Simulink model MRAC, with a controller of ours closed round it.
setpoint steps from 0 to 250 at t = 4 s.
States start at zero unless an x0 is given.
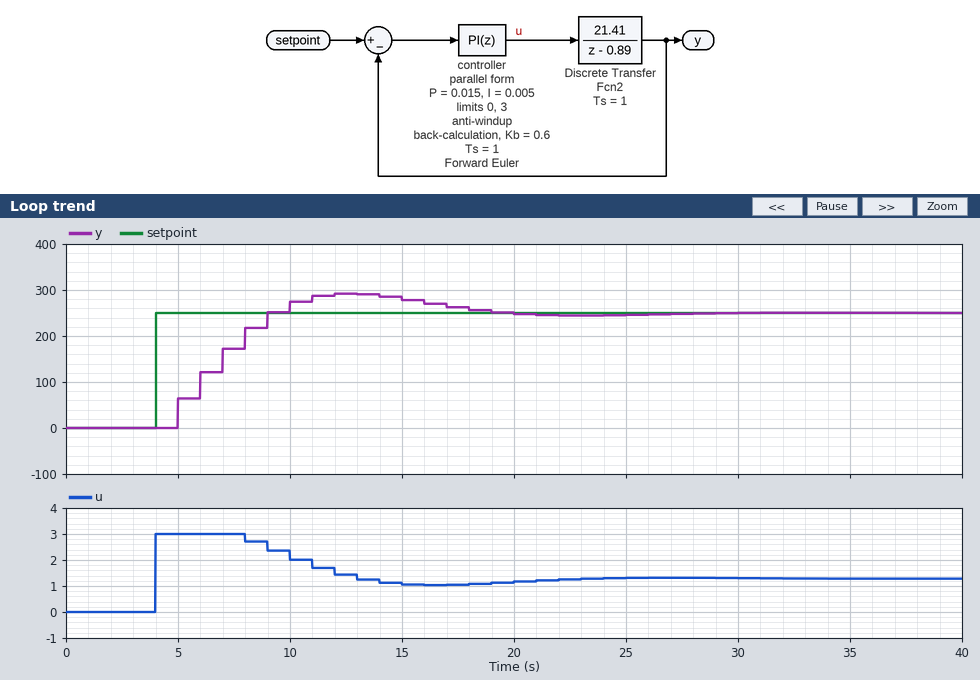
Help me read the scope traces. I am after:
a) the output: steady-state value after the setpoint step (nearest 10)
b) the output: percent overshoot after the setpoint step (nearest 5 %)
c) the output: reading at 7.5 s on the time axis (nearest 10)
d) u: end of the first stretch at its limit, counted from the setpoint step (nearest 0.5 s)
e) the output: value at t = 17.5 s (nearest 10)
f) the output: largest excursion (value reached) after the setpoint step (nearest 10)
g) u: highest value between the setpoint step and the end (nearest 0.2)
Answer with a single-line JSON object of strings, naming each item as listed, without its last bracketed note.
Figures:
{"the output: steady-state value after the setpoint step": "250", "the output: percent overshoot after the setpoint step": "15 %", "the output: reading at 7.5 s on the time axis": "170", "u: end of the first stretch at its limit, counted from the setpoint step": "4.0 s", "the output: value at t = 17.5 s": "260", "the output: largest excursion (value reached) after the setpoint step": "290", "u: highest value between the setpoint step and the end": "3.0"}
